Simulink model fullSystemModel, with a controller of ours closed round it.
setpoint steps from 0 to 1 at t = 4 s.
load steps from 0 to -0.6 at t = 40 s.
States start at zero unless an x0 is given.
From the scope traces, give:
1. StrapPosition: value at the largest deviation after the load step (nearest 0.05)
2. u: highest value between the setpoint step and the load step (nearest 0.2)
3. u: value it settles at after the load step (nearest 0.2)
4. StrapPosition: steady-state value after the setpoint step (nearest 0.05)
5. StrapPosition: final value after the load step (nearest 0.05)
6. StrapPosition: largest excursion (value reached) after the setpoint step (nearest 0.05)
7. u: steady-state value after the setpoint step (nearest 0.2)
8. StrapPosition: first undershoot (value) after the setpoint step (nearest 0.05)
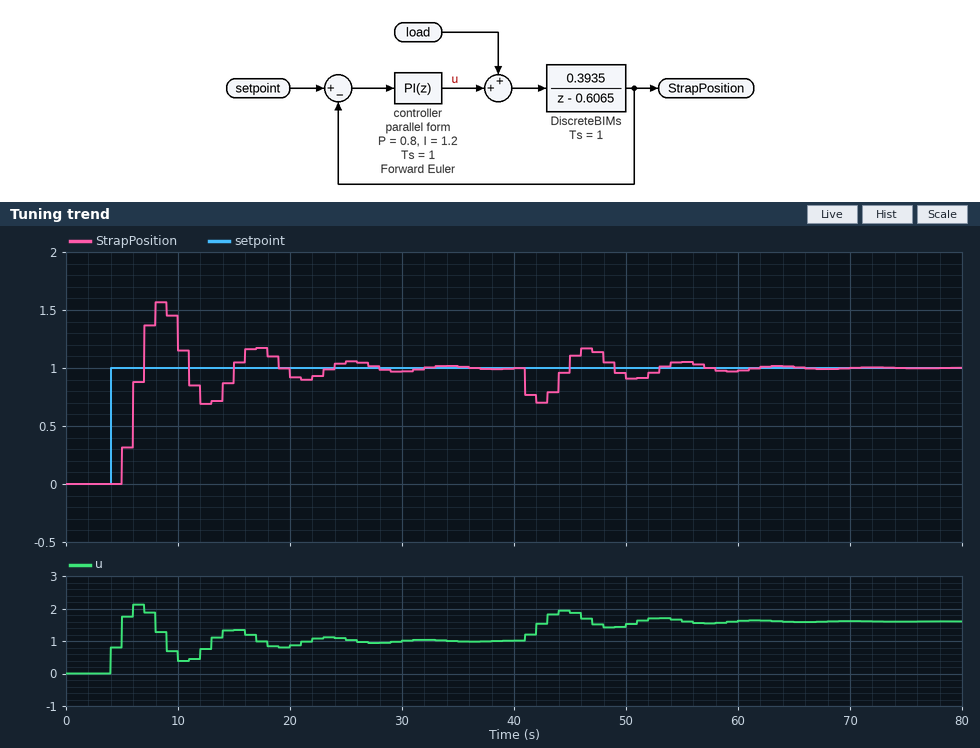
0.70
2.2
1.6
1.00
1.00
1.55
1.0
0.70
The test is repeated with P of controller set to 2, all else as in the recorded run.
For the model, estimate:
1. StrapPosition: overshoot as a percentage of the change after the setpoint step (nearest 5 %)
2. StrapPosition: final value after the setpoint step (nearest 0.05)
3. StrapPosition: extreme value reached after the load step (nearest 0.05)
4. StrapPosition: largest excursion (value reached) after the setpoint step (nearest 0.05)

15 %
1.00
0.75
1.15
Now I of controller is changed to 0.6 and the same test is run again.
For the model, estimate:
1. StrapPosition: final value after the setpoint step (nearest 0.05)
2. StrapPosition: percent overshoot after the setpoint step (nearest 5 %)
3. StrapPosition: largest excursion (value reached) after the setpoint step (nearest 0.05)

1.00
15 %
1.15
